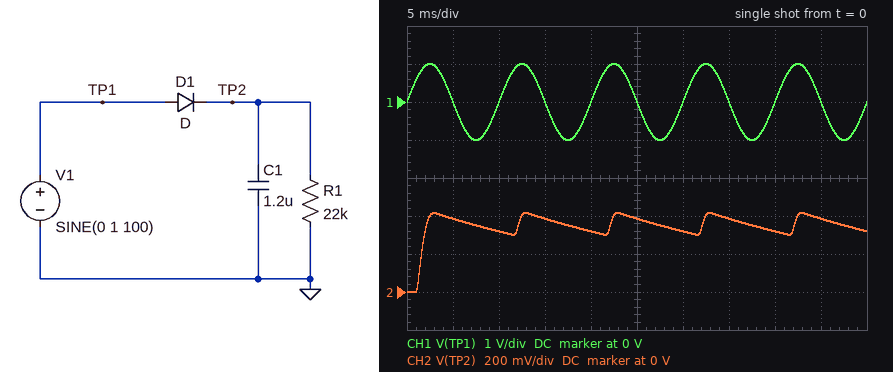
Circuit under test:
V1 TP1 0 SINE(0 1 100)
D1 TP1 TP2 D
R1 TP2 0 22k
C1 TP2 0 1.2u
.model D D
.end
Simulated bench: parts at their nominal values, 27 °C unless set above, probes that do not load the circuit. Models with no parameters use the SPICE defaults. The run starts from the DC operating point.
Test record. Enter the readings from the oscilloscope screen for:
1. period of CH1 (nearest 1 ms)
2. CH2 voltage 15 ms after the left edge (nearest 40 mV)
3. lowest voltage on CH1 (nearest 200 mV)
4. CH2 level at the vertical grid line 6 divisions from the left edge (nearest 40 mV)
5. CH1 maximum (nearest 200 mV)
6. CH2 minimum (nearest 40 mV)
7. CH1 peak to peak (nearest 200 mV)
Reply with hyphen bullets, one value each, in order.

- 10 ms
- 400 mV
- -1.0 V
- 320 mV
- 1.0 V
- 0 V
- 2.0 V
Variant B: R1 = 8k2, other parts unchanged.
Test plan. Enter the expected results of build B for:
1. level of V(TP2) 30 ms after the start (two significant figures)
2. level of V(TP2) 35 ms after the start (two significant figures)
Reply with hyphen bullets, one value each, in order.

- 200 mV
- 330 mV
